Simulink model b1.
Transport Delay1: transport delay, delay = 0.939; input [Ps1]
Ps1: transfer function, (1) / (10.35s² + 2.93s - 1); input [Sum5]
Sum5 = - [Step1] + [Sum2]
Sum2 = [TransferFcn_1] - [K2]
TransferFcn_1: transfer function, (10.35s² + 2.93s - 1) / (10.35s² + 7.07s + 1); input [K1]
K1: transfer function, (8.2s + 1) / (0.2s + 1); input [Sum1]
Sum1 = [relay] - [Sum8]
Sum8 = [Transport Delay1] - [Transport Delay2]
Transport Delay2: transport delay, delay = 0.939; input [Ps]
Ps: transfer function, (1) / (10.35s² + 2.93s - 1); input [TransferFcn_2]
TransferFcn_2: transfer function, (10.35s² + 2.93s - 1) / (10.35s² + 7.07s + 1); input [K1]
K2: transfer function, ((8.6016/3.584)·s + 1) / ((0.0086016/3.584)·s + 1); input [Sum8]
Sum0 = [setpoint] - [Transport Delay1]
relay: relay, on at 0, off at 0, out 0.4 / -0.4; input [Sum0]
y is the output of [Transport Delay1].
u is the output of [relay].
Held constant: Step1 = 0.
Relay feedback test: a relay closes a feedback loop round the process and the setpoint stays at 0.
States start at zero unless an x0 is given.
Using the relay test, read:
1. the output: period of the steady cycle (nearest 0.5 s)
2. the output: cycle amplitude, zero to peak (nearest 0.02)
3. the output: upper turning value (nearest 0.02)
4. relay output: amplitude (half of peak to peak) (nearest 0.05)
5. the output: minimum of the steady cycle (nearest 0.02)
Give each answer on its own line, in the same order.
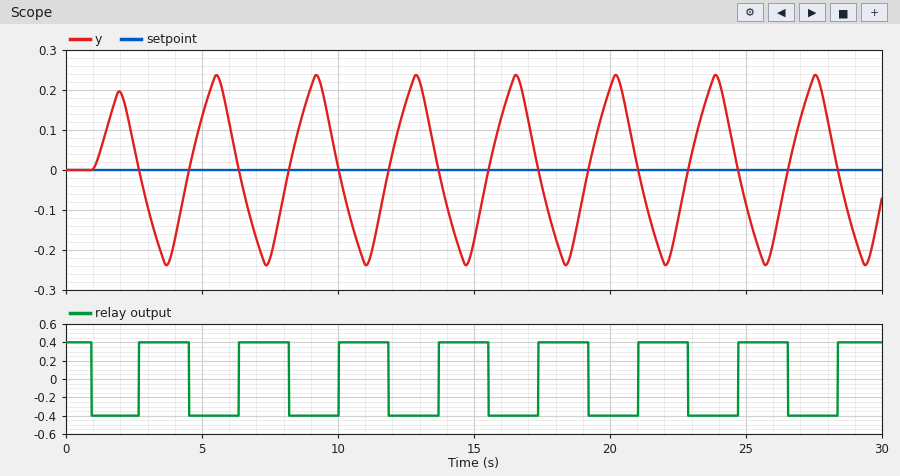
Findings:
3.5 s
0.24
0.24
0.40
-0.24
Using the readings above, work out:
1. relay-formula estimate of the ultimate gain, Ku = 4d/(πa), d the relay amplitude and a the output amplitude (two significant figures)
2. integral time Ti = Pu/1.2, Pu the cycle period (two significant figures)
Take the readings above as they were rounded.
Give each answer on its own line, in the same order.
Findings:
2.1
2.9 s
